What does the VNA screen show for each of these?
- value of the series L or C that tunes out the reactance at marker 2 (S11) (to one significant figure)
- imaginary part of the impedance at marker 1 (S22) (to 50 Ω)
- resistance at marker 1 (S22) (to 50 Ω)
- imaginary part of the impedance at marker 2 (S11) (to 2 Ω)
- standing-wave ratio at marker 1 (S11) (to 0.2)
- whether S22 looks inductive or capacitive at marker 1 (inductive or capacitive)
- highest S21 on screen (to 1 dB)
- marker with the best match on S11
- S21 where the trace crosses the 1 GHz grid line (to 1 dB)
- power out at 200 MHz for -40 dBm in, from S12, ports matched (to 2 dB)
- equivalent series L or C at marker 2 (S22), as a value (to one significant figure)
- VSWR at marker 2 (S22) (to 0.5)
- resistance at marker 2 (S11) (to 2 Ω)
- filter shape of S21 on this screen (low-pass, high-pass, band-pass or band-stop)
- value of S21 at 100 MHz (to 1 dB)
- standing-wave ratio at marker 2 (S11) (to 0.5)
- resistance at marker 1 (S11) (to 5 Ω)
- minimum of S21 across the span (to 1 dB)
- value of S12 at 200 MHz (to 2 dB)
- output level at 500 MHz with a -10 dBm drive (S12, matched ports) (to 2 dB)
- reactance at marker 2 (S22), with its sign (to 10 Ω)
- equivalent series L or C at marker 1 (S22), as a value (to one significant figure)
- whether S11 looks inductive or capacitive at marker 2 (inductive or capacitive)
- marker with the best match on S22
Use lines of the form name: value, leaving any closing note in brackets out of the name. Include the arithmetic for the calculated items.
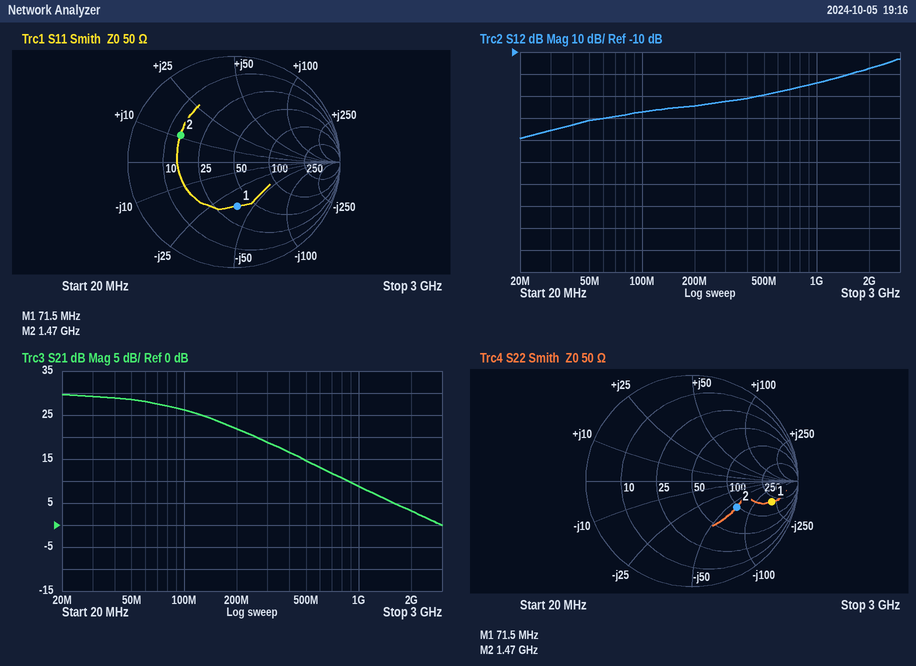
value of the series L or C that tunes out the reactance at marker 2 (S11): C = 1/(2π × 1.47 GHz × 10 Ω) ≈ 10.8 pF, so 10 pF to one significant figure
imaginary part of the impedance at marker 1 (S22): -200 Ω
resistance at marker 1 (S22): 200 Ω
imaginary part of the impedance at marker 2 (S11): +10 Ω
standing-wave ratio at marker 1 (S11): 2.4
whether S22 looks inductive or capacitive at marker 1: capacitive
highest S21 on screen: 30 dB
marker with the best match on S11: marker 1
S21 where the trace crosses the 1 GHz grid line: 9 dB
power out at 200 MHz for -40 dBm in, from S12, ports matched: -40 dBm + (-34 dB) = -74 dBm
equivalent series L or C at marker 2 (S22), as a value: C = 1/(2π × 1.47 GHz × 60 Ω) ≈ 2 pF
VSWR at marker 2 (S22): 3.0
resistance at marker 2 (S11): 14 Ω
filter shape of S21 on this screen: low-pass
value of S21 at 100 MHz: 26 dB
standing-wave ratio at marker 2 (S11): 3.5
resistance at marker 1 (S11): 35 Ω
minimum of S21 across the span: 0 dB
value of S12 at 200 MHz: -34 dB
output level at 500 MHz with a -10 dBm drive (S12, matched ports): -10 dBm + (-30 dB) = -40 dBm
reactance at marker 2 (S22), with its sign: -60 Ω
equivalent series L or C at marker 1 (S22), as a value: C = 1/(2π × 71.5 MHz × 200 Ω) ≈ 11.1 pF, so 10 pF to one significant figure
whether S11 looks inductive or capacitive at marker 2: inductive
marker with the best match on S22: marker 2
